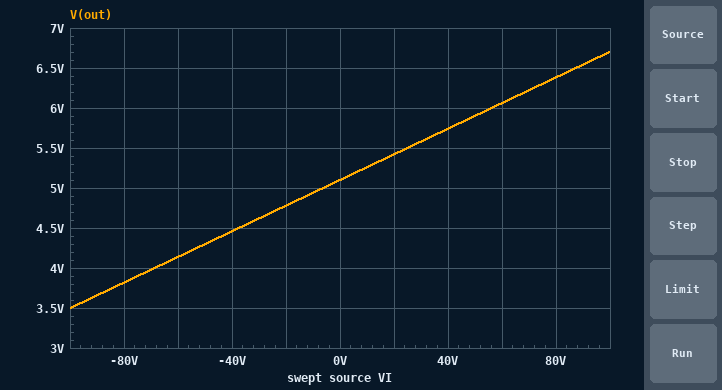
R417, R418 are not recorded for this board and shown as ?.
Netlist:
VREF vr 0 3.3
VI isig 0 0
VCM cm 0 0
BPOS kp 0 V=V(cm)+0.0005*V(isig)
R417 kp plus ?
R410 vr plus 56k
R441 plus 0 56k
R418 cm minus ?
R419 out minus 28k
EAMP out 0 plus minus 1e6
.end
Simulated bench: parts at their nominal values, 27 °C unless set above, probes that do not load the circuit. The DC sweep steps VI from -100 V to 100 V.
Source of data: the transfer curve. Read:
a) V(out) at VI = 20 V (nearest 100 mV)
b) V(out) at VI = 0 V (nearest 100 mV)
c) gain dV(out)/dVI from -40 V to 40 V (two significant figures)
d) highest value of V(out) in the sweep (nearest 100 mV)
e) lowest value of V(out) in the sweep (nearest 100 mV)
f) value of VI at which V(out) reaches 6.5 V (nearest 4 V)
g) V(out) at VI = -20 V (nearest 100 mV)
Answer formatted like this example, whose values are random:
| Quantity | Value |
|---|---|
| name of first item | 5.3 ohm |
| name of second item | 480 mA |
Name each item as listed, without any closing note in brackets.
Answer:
| Quantity | Value |
|---|---|
| V(out) at VI = 20 V | 5.4 V |
| V(out) at VI = 0 V | 5.1 V |
| gain dV(out)/dVI from -40 V to 40 V | 0.016 V/V |
| highest value of V(out) in the sweep | 6.7 V |
| lowest value of V(out) in the sweep | 3.5 V |
| value of VI at which V(out) reaches 6.5 V | 88 V |
| V(out) at VI = -20 V | 4.8 V |
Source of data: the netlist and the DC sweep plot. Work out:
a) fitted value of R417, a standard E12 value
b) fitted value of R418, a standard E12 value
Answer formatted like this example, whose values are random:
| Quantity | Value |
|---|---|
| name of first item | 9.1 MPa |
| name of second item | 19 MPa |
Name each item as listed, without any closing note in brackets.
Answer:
| Quantity | Value |
|---|---|
| fitted value of R417, a standard E12 value | 2.7 kΩ |
| fitted value of R418, a standard E12 value | 820 Ω |
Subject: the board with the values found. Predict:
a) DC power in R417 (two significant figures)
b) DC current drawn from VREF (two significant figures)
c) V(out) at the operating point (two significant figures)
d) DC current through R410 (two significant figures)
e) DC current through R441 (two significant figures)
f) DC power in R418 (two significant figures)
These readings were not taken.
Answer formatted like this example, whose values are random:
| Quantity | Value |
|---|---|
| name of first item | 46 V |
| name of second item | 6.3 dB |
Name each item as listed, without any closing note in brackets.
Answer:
| Quantity | Value |
|---|---|
| DC power in R417 | 7.8 µW |
| DC current drawn from VREF | 56 µA |
| V(out) at the operating point | 5.1 V |
| DC current through R410 | 56 µA |
| DC current through R441 | 2.6 µA |
| DC power in R418 | 26 µW |
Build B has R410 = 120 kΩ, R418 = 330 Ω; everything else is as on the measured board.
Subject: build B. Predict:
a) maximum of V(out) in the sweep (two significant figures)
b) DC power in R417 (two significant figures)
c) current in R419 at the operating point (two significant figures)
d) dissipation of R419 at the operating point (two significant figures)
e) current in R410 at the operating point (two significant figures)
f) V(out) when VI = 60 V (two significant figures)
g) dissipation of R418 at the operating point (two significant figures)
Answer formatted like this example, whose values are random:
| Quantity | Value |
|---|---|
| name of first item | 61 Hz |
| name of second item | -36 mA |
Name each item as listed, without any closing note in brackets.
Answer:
| Quantity | Value |
|---|---|
| maximum of V(out) in the sweep | 10 V |
| DC power in R417 | 1.8 µW |
| current in R419 at the operating point | 210 µA |
| dissipation of R419 at the operating point | 1.2 mW |
| current in R410 at the operating point | 27 µA |
| V(out) when VI = 60 V | 8.4 V |
| dissipation of R418 at the operating point | 15 µW |
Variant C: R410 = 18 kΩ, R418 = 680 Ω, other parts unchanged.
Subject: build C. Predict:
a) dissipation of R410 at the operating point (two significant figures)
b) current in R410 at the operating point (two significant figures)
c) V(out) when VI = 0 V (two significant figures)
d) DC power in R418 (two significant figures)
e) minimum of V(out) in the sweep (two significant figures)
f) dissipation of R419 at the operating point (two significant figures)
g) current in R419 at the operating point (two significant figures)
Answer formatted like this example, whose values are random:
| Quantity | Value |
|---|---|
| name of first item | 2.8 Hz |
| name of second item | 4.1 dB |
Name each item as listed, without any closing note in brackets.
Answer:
| Quantity | Value |
|---|---|
| dissipation of R410 at the operating point | 460 µW |
| current in R410 at the operating point | 160 µA |
| V(out) when VI = 0 V | 17 V |
| DC power in R418 | 250 µW |
| minimum of V(out) in the sweep | 16 V |
| dissipation of R419 at the operating point | 10 mW |
| current in R419 at the operating point | 610 µA |
